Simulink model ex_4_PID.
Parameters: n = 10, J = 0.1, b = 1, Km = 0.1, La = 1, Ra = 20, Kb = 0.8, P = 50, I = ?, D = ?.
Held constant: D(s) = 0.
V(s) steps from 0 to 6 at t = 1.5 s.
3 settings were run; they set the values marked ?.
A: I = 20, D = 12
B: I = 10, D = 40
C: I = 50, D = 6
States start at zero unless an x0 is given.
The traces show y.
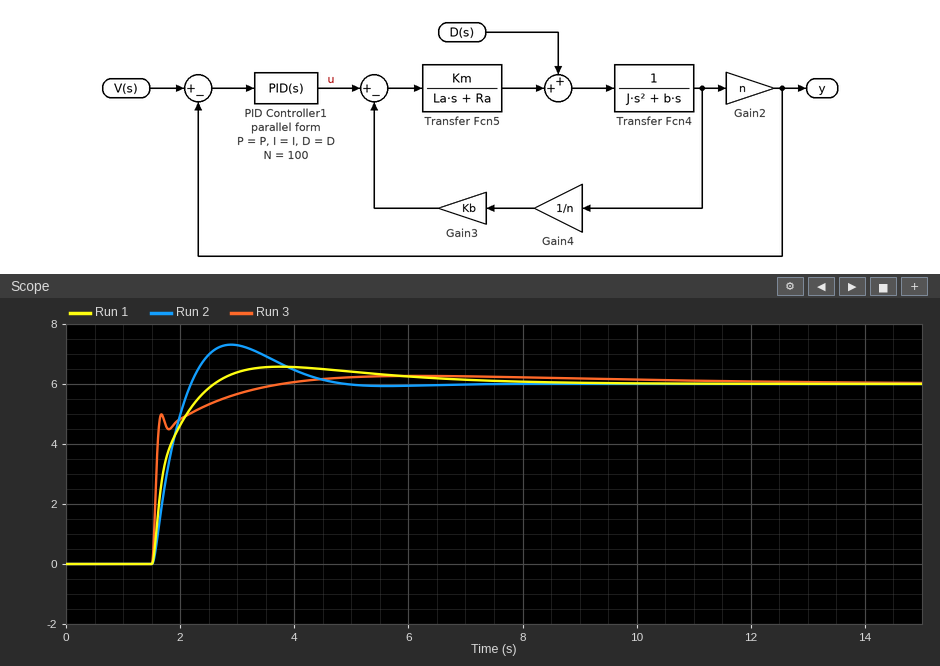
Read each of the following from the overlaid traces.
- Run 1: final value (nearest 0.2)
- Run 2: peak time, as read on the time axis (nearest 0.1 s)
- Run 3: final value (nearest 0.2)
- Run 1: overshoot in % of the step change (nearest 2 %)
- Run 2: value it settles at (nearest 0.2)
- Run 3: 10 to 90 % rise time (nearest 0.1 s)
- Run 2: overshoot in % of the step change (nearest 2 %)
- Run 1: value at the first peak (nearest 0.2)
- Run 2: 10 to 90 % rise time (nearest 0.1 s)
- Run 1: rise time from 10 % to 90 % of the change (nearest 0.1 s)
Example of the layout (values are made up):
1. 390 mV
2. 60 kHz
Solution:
1. 6.0
2. 2.9 s
3. 6.0
4. 10 %
5. 6.0
6. 1.1 s
7. 22 %
8. 6.6
9. 0.5 s
10. 0.7 s
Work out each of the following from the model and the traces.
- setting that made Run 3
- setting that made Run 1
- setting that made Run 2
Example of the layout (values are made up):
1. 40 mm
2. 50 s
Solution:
1. B
2. A
3. C
